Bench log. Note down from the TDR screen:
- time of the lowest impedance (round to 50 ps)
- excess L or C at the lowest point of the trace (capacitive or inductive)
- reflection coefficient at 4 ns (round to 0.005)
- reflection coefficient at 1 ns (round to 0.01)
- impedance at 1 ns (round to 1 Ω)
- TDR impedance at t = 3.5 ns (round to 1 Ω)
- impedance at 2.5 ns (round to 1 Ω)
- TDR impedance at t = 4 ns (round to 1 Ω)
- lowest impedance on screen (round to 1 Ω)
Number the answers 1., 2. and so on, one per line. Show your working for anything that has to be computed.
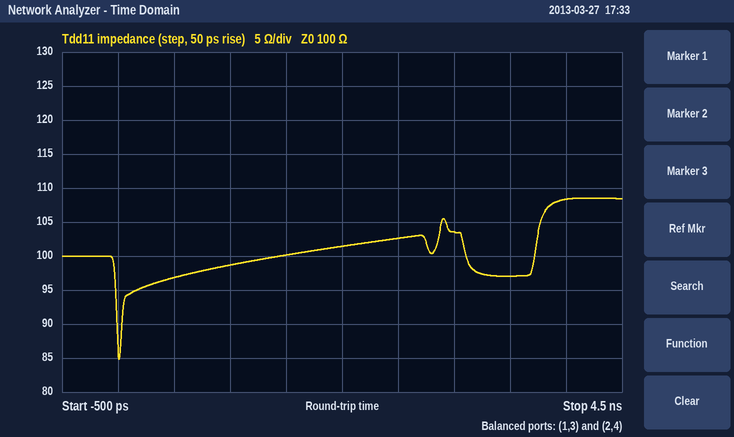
1. 0 ps
2. capacitive
3. (108 − 100)/(108 + 100) ≈ +0.0385, so +0.040 to the nearest 0.005
4. (99 − 100)/(99 + 100) ≈ -0.01
5. 99 Ω
6. 97 Ω
7. 103 Ω
8. 108 Ω
9. 85 Ω
